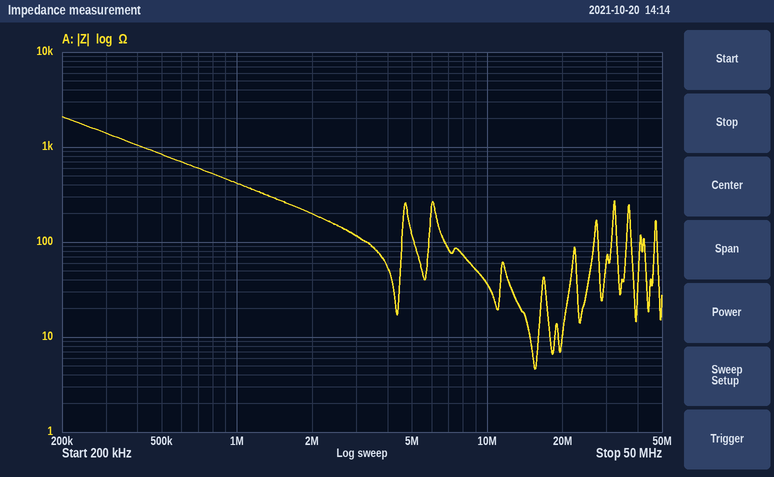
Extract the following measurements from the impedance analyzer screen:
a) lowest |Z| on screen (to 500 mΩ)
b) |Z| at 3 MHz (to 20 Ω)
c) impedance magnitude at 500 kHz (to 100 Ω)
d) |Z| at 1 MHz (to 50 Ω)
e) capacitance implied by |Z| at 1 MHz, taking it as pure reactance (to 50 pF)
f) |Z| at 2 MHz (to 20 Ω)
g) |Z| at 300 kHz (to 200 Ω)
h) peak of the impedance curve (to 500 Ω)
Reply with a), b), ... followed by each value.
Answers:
a) 4.5 Ω
b) 120 Ω
c) 800 Ω
d) 400 Ω
e) 400 pF
f) 200 Ω
g) 1.4 kΩ
h) 2.0 kΩ
